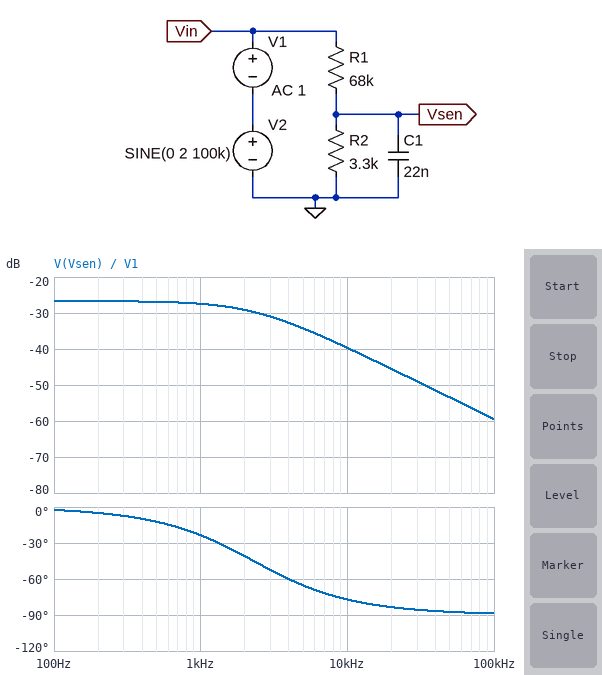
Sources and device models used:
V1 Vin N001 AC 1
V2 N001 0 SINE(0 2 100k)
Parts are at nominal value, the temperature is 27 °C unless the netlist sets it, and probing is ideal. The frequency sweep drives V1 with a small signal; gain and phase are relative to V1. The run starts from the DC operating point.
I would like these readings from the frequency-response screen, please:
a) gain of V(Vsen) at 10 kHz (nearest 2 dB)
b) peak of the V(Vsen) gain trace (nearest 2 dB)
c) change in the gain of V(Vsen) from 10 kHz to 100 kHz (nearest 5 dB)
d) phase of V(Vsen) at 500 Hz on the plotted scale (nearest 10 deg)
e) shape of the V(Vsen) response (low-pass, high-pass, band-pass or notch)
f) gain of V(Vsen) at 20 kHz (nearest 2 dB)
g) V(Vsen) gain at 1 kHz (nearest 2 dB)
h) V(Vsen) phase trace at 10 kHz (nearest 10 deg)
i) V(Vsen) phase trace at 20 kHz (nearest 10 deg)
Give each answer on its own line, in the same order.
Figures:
-40 dB
-26 dB
-20 dB
-10 deg
low-pass
-46 dB
-28 dB
-80 deg
-80 deg
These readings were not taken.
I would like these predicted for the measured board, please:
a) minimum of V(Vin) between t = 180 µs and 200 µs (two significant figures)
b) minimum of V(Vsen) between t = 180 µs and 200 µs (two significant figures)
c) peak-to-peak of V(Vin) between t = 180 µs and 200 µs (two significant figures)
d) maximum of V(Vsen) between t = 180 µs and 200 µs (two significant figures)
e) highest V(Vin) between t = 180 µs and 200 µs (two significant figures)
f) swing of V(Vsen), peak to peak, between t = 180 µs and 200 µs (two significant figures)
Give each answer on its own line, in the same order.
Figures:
-2.0 V
-2.0 mV
4.0 V
2.3 mV
2.0 V
4.3 mV
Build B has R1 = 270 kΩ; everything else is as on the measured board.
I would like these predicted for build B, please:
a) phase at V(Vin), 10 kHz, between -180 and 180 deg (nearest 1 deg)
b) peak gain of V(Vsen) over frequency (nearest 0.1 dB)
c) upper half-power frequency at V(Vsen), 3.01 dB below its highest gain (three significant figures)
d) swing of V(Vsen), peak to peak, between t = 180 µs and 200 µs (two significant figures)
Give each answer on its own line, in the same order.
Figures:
0 deg
-38.4 dB
2.22 kHz
1.1 mV
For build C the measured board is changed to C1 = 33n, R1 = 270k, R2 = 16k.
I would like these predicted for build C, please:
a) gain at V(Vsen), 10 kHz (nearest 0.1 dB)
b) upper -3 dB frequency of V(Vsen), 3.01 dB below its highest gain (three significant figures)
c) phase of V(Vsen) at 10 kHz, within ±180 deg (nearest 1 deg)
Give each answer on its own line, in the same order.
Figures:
-55.0 dB
319 Hz
-88 deg
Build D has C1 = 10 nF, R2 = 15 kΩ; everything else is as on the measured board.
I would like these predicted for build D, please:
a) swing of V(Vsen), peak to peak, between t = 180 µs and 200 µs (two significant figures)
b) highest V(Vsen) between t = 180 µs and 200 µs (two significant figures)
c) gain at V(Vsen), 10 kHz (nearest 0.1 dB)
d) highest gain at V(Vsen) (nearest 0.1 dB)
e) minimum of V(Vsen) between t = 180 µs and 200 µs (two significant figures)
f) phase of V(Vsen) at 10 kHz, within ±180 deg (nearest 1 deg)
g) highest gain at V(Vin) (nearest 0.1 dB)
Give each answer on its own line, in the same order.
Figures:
9.5 mV
5.7 mV
-32.7 dB
-14.9 dB
-3.8 mV
-83 deg
0 dB
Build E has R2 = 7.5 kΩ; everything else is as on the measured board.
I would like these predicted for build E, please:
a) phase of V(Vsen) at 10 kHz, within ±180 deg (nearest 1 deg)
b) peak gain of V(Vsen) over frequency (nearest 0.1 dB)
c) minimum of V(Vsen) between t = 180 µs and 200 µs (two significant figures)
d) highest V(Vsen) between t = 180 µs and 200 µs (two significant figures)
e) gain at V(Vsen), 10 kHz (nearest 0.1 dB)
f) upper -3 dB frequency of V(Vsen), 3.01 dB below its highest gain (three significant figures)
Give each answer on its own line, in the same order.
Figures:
-84 deg
-20.1 dB
-1.6 mV
2.7 mV
-39.5 dB
1.07 kHz
